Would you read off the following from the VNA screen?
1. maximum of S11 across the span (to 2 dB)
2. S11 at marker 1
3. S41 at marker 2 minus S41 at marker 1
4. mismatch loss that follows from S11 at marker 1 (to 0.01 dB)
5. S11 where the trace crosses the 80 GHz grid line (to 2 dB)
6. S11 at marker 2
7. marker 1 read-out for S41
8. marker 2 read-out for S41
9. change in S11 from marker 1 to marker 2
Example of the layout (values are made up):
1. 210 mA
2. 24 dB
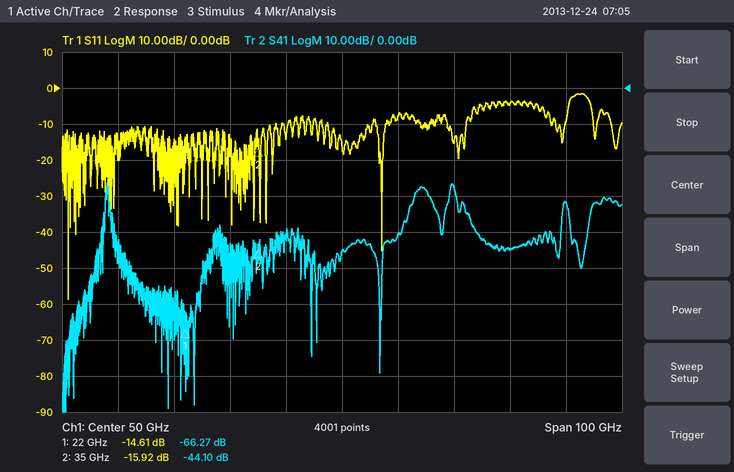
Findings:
1. -2 dB
2. -14.61 dB
3. 22.17 dB
4. 0.15 dB
5. -4 dB
6. -15.92 dB
7. -66.27 dB
8. -44.10 dB
9. -1.31 dB
